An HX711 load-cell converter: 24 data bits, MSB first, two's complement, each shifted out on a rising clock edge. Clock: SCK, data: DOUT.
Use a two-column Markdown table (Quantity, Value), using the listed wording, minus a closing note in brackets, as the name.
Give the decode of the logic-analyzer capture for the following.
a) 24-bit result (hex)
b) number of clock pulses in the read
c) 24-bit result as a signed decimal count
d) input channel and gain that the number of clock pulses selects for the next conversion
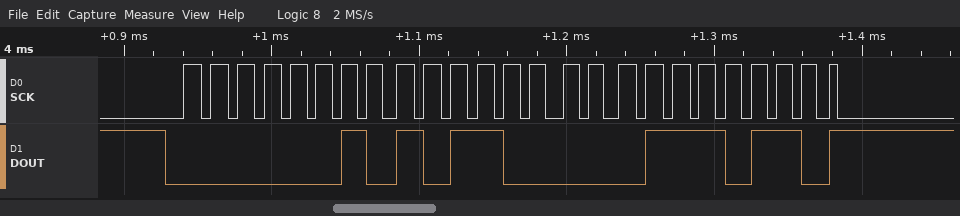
| Quantity | Value |
|---|---|
| 24-bit result | 0x02B076 |
| number of clock pulses in the read | 25 |
| 24-bit result as a signed decimal count | 176246 |
| input channel and gain that the number of clock pulses selects for the next conversion | channel A, gain 128 |
